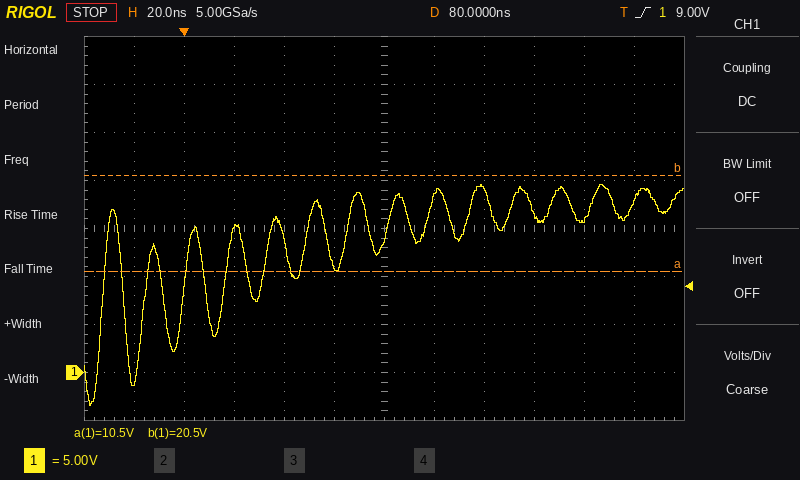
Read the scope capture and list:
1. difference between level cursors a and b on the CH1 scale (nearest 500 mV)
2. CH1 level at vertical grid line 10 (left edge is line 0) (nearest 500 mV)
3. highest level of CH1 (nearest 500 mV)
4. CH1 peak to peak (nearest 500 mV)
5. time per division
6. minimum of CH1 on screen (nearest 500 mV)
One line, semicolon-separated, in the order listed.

10.0 V; 16.0 V; 19.5 V; 23.0 V; 20 ns; -3.5 V
